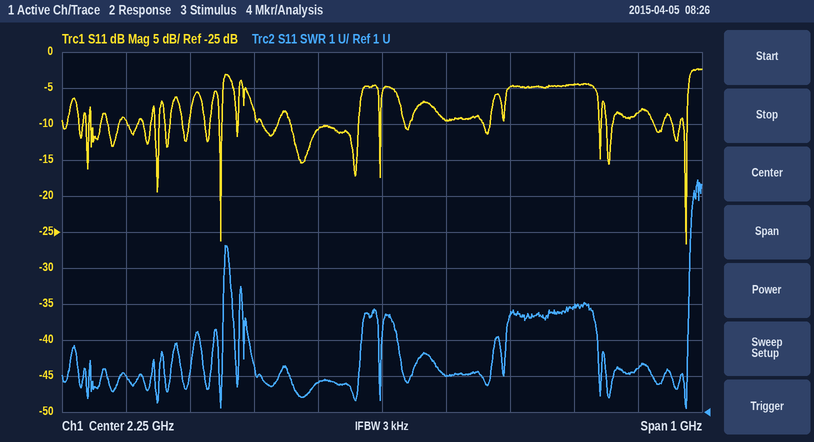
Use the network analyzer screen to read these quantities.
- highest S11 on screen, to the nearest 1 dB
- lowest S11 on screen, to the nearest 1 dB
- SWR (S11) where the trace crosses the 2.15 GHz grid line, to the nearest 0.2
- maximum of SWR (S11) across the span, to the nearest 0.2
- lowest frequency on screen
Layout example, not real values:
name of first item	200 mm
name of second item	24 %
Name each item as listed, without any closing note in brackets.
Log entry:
highest S11 on screen, to the nearest 1 dB	-2 dB
lowest S11 on screen, to the nearest 1 dB	-27 dB
SWR (S11) where the trace crosses the 2.15 GHz grid line, to the nearest 0.2	1.8
maximum of SWR (S11) across the span, to the nearest 0.2	7.4
lowest frequency on screen	1.75 GHz
